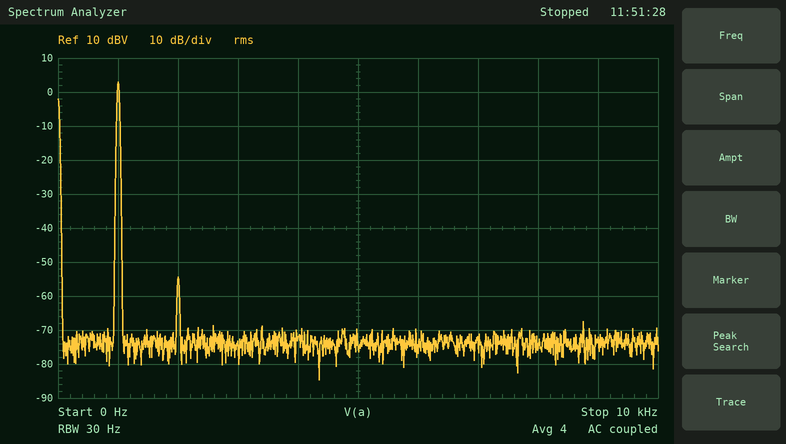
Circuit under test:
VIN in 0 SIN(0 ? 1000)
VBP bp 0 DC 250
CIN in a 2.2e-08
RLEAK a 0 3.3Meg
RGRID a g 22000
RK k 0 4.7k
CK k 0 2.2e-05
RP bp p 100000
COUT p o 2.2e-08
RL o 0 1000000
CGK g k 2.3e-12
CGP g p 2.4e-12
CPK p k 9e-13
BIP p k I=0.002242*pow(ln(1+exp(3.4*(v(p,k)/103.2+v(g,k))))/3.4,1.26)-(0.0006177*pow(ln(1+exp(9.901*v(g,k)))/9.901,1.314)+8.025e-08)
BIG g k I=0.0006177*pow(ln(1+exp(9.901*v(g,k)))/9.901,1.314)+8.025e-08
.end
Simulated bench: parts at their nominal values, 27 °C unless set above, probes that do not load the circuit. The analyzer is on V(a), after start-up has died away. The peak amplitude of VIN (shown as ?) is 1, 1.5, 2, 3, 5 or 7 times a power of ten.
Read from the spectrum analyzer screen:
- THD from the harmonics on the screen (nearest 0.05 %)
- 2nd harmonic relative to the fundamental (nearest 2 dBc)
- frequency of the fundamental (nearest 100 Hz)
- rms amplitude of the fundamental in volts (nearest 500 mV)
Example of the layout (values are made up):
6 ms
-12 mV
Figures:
0.15 %
-58 dBc
1.0 kHz
1.5 V
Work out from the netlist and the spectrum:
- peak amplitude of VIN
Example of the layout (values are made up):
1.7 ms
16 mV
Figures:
2 V
